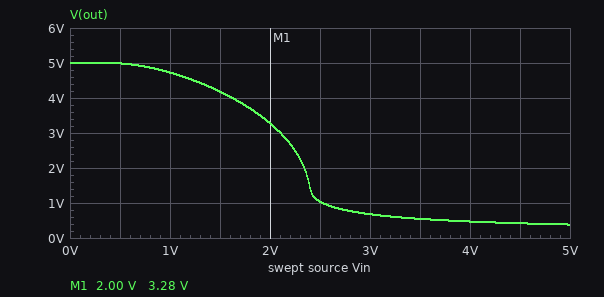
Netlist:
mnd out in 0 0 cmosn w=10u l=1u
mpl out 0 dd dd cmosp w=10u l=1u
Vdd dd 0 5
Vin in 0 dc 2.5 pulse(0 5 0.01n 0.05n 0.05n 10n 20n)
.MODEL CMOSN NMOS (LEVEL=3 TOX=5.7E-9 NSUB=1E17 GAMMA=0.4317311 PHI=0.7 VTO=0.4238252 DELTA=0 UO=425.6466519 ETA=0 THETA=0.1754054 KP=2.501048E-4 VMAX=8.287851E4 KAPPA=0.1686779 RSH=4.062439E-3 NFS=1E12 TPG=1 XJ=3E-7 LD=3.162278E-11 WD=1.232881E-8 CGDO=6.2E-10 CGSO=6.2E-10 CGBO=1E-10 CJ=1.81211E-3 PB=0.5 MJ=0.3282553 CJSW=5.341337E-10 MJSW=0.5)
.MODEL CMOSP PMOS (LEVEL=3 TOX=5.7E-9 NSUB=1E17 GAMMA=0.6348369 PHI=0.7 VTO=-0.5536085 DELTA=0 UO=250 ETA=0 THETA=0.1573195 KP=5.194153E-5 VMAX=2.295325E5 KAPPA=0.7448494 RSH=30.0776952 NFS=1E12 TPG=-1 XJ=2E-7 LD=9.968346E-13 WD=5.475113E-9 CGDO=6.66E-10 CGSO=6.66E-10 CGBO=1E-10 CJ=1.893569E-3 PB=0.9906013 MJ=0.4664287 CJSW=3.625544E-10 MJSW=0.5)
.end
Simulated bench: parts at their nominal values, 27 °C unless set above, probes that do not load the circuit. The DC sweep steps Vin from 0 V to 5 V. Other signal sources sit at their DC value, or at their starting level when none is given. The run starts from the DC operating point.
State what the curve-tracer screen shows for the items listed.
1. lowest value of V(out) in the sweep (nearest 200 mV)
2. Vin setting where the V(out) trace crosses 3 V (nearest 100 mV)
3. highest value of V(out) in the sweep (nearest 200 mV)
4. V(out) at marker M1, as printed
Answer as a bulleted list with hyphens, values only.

- 400 mV
- 2.1 V
- 5.0 V
- 3.28 V
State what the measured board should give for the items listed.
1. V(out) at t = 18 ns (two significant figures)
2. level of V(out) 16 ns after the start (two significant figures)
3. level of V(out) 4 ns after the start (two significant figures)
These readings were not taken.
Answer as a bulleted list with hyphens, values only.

- 5.0 V
- 5.0 V
- 380 mV
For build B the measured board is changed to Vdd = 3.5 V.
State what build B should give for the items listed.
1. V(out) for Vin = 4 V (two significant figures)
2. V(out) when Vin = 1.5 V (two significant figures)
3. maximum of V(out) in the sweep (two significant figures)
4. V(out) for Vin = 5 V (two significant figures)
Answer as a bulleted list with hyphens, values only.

- 230 mV
- 2.3 V
- 3.5 V
- 190 mV
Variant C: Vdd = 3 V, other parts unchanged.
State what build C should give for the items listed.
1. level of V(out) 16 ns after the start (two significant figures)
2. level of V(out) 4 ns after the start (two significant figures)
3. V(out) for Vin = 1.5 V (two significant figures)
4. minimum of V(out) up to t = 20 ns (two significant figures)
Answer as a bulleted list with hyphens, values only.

- 3.0 V
- 140 mV
- 970 mV
- -690 mV
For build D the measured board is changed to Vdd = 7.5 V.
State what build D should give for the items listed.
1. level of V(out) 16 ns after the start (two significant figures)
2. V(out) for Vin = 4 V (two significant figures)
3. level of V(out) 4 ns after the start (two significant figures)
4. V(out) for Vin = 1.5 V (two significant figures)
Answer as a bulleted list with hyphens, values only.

- 7.5 V
- 1.2 V
- 870 mV
- 6.9 V
